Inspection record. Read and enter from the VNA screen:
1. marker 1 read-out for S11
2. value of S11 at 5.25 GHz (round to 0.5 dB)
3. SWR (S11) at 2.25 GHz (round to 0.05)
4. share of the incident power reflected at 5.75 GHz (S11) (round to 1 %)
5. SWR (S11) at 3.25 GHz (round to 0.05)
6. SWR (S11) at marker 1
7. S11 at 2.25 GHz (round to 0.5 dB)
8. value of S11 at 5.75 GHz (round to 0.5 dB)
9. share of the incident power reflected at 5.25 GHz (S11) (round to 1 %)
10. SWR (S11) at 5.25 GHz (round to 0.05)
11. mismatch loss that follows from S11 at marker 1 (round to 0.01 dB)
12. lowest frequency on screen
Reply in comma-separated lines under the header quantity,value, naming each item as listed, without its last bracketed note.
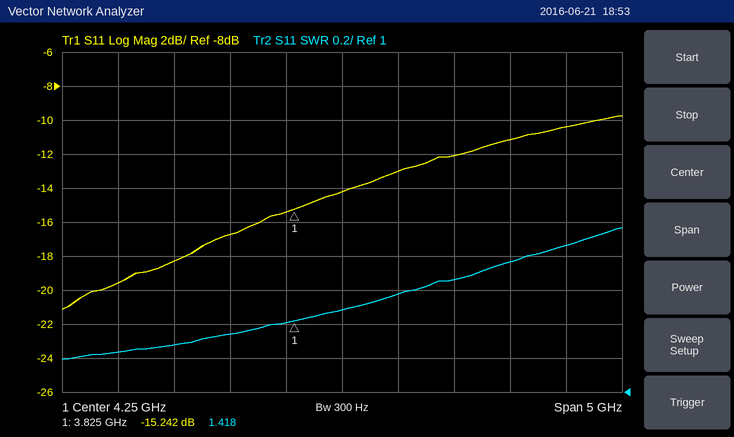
quantity,value
marker 1 read-out for S11,-15.242 dB
value of S11 at 5.25 GHz,-12.0 dB
SWR (S11) at 2.25 GHz,1.25
share of the incident power reflected at 5.75 GHz (S11),8 %
SWR (S11) at 3.25 GHz,1.35
SWR (S11) at marker 1,1.418
S11 at 2.25 GHz,-19.5 dB
value of S11 at 5.75 GHz,-11.0 dB
share of the incident power reflected at 5.25 GHz (S11),6 %
SWR (S11) at 5.25 GHz,1.65
mismatch loss that follows from S11 at marker 1,0.13 dB
lowest frequency on screen,1.75 GHz
